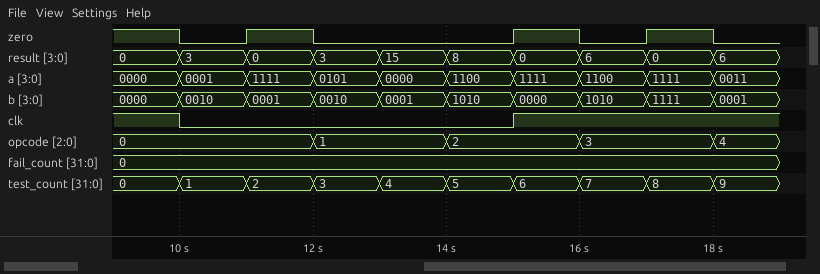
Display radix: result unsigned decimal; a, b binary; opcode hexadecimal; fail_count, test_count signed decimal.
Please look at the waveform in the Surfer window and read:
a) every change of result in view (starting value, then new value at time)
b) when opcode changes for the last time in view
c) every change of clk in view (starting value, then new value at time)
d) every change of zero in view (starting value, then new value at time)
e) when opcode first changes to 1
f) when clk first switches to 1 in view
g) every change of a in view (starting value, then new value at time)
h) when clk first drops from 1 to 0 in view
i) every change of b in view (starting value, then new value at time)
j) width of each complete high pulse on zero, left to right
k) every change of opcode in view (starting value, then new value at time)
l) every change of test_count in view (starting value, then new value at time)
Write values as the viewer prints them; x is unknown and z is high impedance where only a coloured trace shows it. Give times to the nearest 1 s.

0, 3 at 10 s, 0 at 11 s, 3 at 12 s, 15 at 13 s, 8 at 14 s, 0 at 15 s, 6 at 16 s, 0 at 17 s, 6 at 18 s
18 s
1, 0 at 10 s, 1 at 15 s
1, 0 at 10 s, 1 at 11 s, 0 at 12 s, 1 at 15 s, 0 at 16 s, 1 at 17 s, 0 at 18 s
12 s
15 s
0000, 0001 at 10 s, 1111 at 11 s, 0101 at 12 s, 0000 at 13 s, 1100 at 14 s, 1111 at 15 s, 1100 at 16 s, 1111 at 17 s, 0011 at 18 s
10 s
0000, 0010 at 10 s, 0001 at 11 s, 0010 at 12 s, 0001 at 13 s, 1010 at 14 s, 0000 at 15 s, 1010 at 16 s, 1111 at 17 s, 0001 at 18 s
1 s, 1 s, 1 s
0, 1 at 12 s, 2 at 14 s, 3 at 16 s, 4 at 18 s
0, 1 at 10 s, 2 at 11 s, 3 at 12 s, 4 at 13 s, 5 at 14 s, 6 at 15 s, 7 at 16 s, 8 at 17 s, 9 at 18 s
